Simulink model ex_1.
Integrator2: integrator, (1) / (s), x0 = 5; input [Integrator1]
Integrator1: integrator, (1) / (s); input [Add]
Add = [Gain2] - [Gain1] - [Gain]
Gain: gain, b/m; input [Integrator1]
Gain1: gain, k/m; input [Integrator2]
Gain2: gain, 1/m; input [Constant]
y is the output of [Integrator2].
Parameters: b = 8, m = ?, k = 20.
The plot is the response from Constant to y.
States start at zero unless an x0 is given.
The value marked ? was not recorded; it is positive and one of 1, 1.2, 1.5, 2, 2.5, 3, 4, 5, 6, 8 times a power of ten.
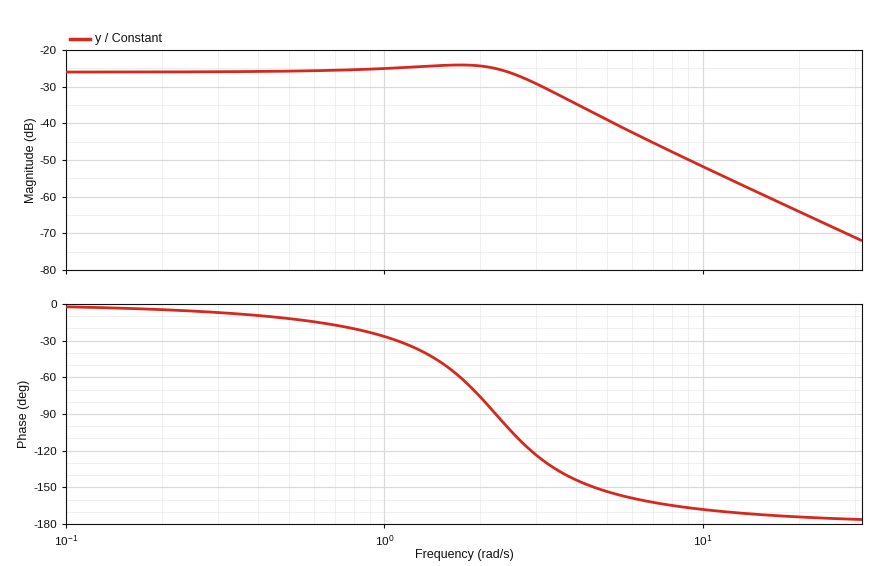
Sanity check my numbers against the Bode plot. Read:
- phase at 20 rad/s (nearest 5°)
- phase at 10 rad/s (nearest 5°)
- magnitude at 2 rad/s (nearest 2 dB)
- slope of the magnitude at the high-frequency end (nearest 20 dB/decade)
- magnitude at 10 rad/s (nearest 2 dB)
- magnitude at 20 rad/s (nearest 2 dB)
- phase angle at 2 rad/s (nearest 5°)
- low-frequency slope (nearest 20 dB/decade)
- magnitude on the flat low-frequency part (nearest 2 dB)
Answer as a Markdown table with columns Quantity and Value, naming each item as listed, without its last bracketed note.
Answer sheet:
| Quantity | Value |
|---|---|
| phase at 20 rad/s | -175° |
| phase at 10 rad/s | -170° |
| magnitude at 2 rad/s | -24 dB |
| slope of the magnitude at the high-frequency end | -40 dB/decade |
| magnitude at 10 rad/s | -52 dB |
| magnitude at 20 rad/s | -64 dB |
| phase angle at 2 rad/s | -75° |
| low-frequency slope | 0 dB/decade |
| magnitude on the flat low-frequency part | -26 dB |
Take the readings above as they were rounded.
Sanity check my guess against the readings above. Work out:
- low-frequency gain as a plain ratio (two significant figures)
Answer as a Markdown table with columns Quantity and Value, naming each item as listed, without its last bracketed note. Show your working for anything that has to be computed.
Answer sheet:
| Quantity | Value |
|---|---|
| low-frequency gain as a plain ratio | 10^(-26 / 20) = 0.050 |
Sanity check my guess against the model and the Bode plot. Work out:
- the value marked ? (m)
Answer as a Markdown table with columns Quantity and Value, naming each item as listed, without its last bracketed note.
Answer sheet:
| Quantity | Value |
|---|---|
| the value marked ? | 4 |
